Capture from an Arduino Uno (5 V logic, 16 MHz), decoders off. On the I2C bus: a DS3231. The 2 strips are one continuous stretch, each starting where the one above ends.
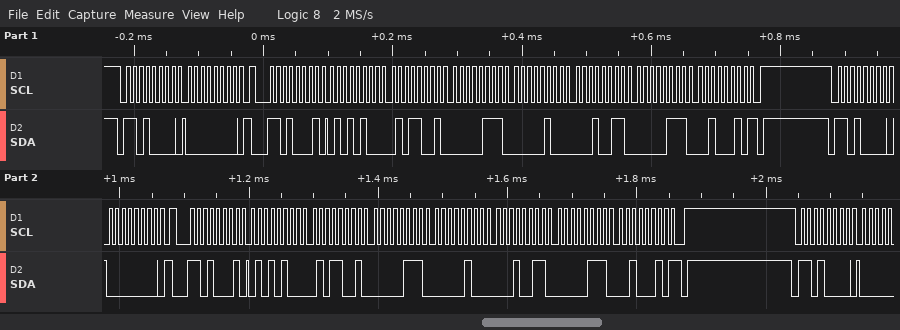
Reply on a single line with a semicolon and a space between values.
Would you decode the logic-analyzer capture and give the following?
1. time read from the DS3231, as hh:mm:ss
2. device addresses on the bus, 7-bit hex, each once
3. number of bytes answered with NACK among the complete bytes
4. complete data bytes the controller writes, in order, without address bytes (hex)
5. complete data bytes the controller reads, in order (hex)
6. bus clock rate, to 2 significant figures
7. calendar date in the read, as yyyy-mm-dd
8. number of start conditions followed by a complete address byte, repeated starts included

07:59:54; 0x68; 2; 00 00; 54 59 07 04 13 07 22 54 59 07 04 13 07 22; 100 kHz; 2022-07-13; 5
